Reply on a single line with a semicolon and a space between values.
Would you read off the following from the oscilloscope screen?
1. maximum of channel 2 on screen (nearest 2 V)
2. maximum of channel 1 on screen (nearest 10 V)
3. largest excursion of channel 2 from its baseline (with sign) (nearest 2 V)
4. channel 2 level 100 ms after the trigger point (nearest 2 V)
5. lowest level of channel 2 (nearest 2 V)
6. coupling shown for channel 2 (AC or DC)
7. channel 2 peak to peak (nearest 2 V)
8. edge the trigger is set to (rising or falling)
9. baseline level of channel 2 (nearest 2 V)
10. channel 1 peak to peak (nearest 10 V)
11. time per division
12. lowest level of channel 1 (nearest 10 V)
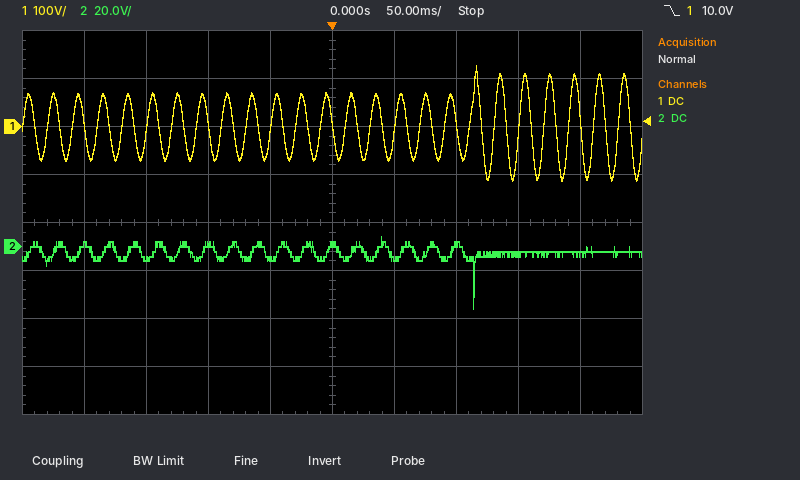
4 V; 130 V; -24 V; 0 V; -26 V; DC; 30 V; falling; -2 V; 240 V; 50 ms; -110 V
